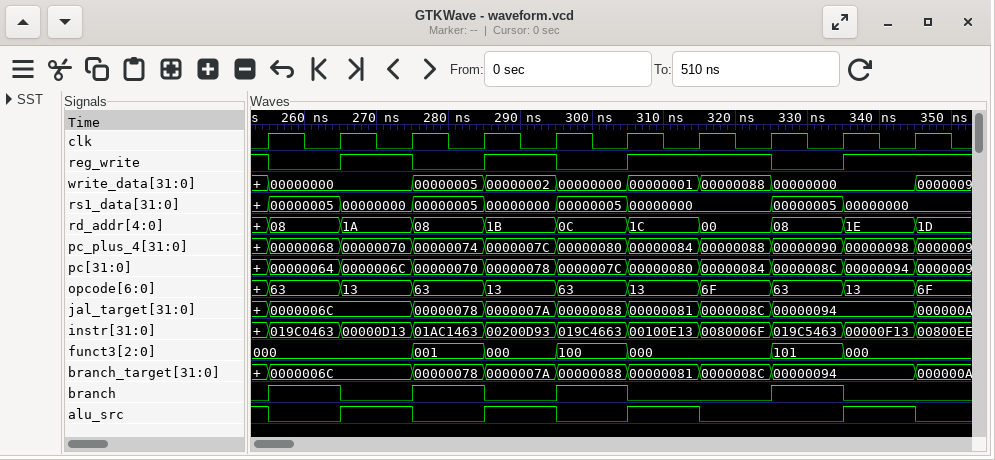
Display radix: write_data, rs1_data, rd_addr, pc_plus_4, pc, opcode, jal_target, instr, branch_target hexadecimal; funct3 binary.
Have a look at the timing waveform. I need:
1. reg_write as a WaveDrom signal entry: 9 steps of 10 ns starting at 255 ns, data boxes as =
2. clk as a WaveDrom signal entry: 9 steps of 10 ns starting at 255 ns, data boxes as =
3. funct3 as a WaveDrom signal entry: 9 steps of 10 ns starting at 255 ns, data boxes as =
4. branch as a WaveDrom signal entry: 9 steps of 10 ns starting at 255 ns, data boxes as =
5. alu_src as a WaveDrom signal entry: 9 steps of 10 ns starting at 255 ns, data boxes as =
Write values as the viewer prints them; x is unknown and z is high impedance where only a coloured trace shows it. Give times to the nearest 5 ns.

{name: 'reg_write', wave: '010101.01'}
{name: 'clk', wave: 'p........'}
{name: 'funct3', wave: '=.====.==', data: '000 001 000 100 000 101 000'}
{name: 'branch', wave: '101010.10'}
{name: 'alu_src', wave: '0101010.1'}
